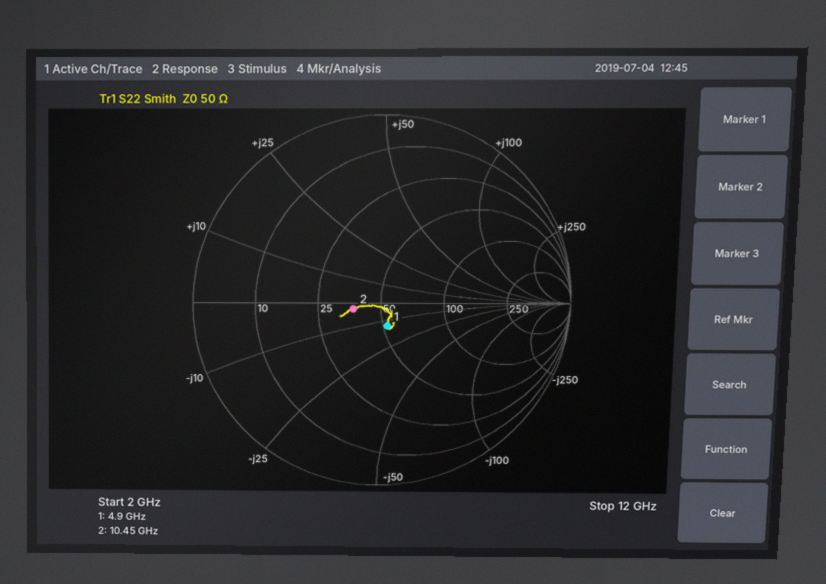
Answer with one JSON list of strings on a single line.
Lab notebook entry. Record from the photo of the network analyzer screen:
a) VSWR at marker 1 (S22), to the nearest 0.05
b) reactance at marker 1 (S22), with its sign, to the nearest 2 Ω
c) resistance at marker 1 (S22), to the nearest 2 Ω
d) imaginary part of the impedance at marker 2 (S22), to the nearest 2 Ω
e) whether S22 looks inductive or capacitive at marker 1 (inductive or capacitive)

["1.30", "-14 Ω", "52 Ω", "-2 Ω", "capacitive"]
